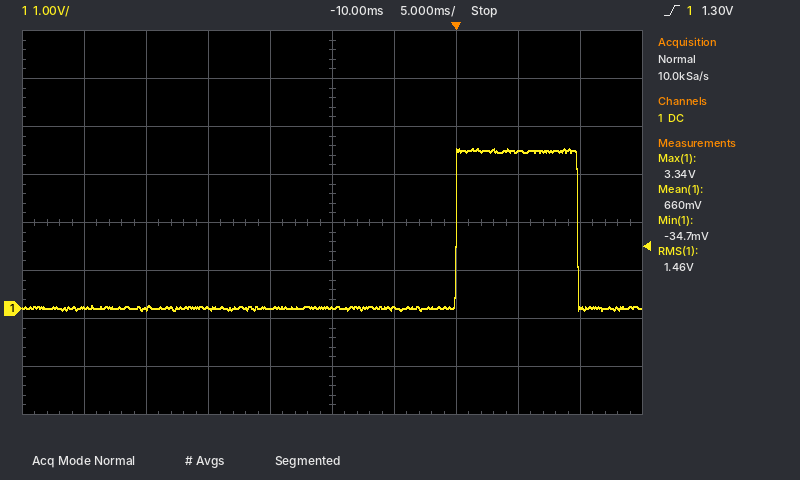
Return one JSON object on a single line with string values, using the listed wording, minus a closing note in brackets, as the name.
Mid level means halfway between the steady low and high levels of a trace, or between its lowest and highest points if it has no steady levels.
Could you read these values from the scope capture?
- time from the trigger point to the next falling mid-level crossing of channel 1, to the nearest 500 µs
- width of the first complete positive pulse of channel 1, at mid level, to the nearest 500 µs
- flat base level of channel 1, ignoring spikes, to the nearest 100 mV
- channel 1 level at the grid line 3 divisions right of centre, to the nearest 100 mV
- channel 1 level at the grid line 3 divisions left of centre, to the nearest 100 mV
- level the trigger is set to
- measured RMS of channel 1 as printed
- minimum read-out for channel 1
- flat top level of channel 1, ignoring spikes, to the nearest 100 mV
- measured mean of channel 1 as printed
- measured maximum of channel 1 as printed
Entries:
{"time from the trigger point to the next falling mid-level crossing of channel 1, to the nearest 500 µs": "10.0 ms", "width of the first complete positive pulse of channel 1, at mid level, to the nearest 500 µs": "10.0 ms", "flat base level of channel 1, ignoring spikes, to the nearest 100 mV": "0.0 V", "channel 1 level at the grid line 3 divisions right of centre, to the nearest 100 mV": "3.3 V", "channel 1 level at the grid line 3 divisions left of centre, to the nearest 100 mV": "0.0 V", "level the trigger is set to": "1.30 V", "measured RMS of channel 1 as printed": "1.46 V", "minimum read-out for channel 1": "-34.7 mV", "flat top level of channel 1, ignoring spikes, to the nearest 100 mV": "3.3 V", "measured mean of channel 1 as printed": "660 mV", "measured maximum of channel 1 as printed": "3.34 V"}
